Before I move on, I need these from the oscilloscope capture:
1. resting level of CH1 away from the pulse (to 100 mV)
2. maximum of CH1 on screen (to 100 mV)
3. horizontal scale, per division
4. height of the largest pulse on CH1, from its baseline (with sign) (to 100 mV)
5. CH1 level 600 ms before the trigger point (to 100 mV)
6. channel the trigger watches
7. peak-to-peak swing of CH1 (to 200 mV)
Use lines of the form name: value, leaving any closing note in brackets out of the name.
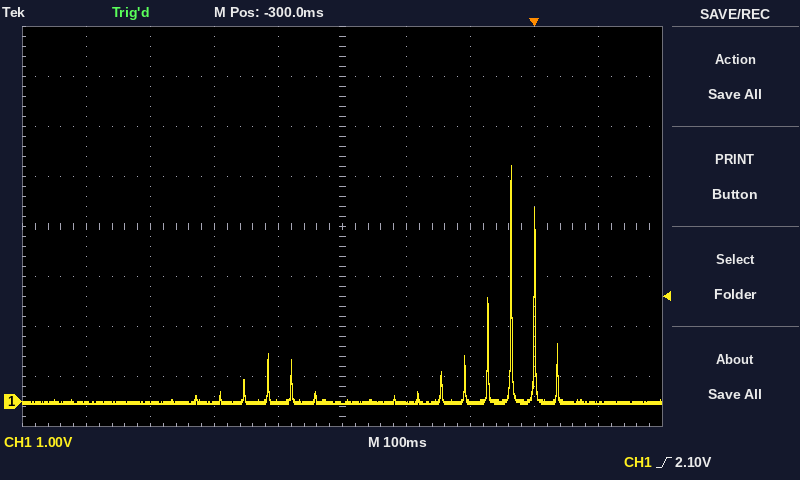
resting level of CH1 away from the pulse: 0.0 V
maximum of CH1 on screen: 4.7 V
horizontal scale, per division: 100 ms
height of the largest pulse on CH1, from its baseline (with sign): +4.7 V
CH1 level 600 ms before the trigger point: 0.0 V
channel the trigger watches: CH1
peak-to-peak swing of CH1: 4.8 V
